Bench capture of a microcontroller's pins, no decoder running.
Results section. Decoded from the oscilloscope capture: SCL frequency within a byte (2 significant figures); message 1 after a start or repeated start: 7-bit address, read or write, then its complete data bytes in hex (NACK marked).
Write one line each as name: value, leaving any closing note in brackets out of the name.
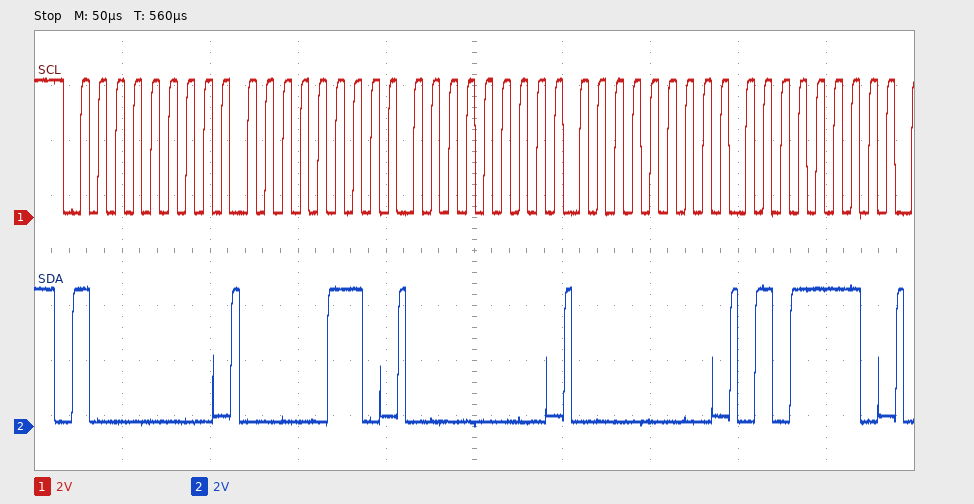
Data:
SCL frequency within a byte: 100 kHz
message 1 after a start or repeated start: 7-bit address, read or write, then its complete data bytes in hex: 0x40 write: 06 00 00 5E
